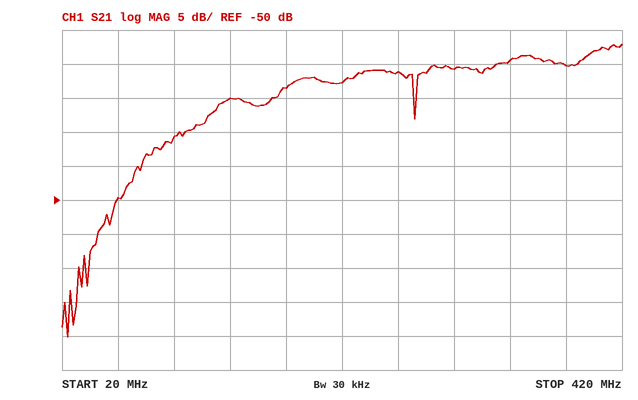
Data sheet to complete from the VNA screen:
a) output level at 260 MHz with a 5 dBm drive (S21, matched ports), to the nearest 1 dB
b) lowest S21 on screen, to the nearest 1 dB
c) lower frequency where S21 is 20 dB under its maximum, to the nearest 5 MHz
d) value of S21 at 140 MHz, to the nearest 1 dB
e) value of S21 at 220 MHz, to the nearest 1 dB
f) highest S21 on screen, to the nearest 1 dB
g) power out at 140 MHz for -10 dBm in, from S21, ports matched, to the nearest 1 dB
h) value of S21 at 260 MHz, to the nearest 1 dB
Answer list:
-26 dBm
-70 dB
70 MHz
-35 dB
-33 dB
-27 dB
-45 dBm
-31 dB
